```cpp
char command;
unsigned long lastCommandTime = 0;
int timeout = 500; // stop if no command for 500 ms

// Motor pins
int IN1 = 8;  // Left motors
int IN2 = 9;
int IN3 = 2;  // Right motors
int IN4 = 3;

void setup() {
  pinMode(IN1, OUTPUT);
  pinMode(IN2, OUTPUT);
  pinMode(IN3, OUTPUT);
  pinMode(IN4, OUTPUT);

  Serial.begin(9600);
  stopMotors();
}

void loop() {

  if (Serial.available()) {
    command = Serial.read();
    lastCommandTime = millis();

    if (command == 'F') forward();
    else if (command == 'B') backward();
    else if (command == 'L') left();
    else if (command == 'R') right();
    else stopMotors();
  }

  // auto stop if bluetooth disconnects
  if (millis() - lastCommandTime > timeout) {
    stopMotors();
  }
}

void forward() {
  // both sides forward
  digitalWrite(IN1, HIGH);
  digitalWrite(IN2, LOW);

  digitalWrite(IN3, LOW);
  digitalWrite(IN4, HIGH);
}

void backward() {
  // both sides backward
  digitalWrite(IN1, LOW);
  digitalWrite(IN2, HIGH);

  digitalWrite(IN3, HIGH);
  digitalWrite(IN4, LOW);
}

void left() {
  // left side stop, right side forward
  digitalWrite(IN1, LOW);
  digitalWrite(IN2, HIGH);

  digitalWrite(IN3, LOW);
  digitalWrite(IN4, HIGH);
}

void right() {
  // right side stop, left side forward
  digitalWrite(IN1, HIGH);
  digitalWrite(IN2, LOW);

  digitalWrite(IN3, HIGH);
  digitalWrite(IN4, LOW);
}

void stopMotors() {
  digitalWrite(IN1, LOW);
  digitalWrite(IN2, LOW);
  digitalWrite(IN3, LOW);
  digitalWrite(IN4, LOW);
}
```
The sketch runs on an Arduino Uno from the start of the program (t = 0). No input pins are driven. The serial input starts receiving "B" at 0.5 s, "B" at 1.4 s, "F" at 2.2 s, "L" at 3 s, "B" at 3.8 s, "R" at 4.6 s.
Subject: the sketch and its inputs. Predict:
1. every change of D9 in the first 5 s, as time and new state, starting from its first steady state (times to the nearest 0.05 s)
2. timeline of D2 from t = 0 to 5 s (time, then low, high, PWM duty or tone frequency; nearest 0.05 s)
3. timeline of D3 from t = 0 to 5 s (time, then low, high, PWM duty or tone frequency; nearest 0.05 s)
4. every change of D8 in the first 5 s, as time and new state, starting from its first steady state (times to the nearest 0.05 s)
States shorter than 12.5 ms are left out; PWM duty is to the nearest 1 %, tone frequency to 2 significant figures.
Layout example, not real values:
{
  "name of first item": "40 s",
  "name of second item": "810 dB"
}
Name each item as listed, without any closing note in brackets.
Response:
{
  "every change of D9 in the first 5 s, as time and new state, starting from its first steady state": "0 s low; 0.5 s high; 1 s low; 1.4 s high; 1.9 s low; 3 s high; 3.5 s low; 3.8 s high; 4.3 s low",
  "timeline of D2 from t = 0 to 5 s": "0 s low; 0.5 s high; 1 s low; 1.4 s high; 1.9 s low; 3.8 s high; 4.3 s low; 4.6 s high",
  "timeline of D3 from t = 0 to 5 s": "0 s low; 2.2 s high; 2.7 s low; 3 s high; 3.5 s low",
  "every change of D8 in the first 5 s, as time and new state, starting from its first steady state": "0 s low; 2.2 s high; 2.7 s low; 4.6 s high"
}
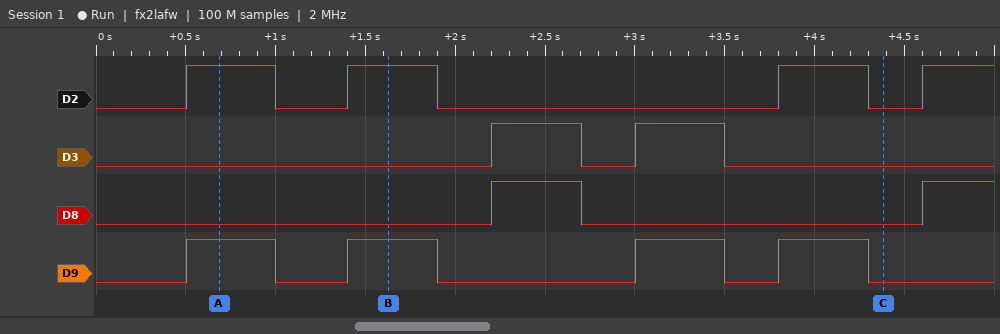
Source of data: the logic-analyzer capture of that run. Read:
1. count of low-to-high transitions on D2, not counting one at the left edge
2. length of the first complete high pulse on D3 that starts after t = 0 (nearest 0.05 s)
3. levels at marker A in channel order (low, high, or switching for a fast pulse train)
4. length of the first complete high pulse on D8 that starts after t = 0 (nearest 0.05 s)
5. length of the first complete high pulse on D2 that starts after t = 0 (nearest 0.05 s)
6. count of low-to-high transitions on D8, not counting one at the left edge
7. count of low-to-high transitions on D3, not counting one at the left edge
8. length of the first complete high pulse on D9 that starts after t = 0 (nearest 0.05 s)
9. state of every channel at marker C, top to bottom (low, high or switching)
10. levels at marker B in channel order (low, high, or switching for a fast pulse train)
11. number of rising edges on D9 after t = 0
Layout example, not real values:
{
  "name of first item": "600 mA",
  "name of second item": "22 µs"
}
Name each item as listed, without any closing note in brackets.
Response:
{
  "count of low-to-high transitions on D2, not counting one at the left edge": "4",
  "length of the first complete high pulse on D3 that starts after t = 0": "0.50 s",
  "levels at marker A in channel order": "D2 high, D3 low, D8 low, D9 high",
  "length of the first complete high pulse on D8 that starts after t = 0": "0.50 s",
  "length of the first complete high pulse on D2 that starts after t = 0": "0.50 s",
  "count of low-to-high transitions on D8, not counting one at the left edge": "2",
  "count of low-to-high transitions on D3, not counting one at the left edge": "2",
  "length of the first complete high pulse on D9 that starts after t = 0": "0.50 s",
  "state of every channel at marker C, top to bottom": "D2 low, D3 low, D8 low, D9 low",
  "levels at marker B in channel order": "D2 high, D3 low, D8 low, D9 high",
  "number of rising edges on D9 after t = 0": "4"
}
